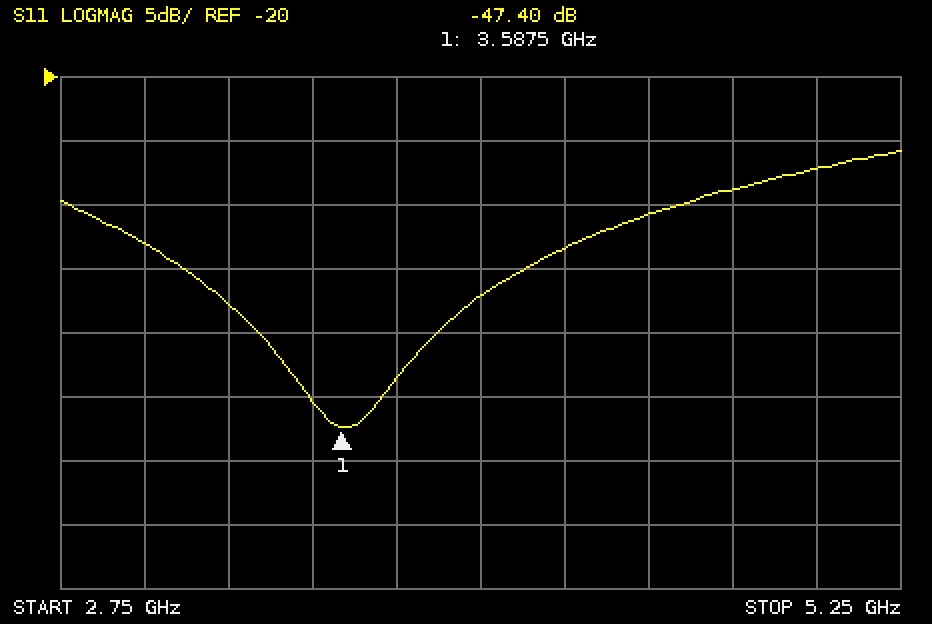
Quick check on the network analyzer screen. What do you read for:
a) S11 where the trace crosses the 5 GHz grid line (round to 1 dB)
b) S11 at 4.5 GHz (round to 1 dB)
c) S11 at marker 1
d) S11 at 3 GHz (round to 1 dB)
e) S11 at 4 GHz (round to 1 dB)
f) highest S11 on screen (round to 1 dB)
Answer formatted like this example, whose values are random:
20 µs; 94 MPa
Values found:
-27 dB; -31 dB; -47.40 dB; -33 dB; -37 dB; -26 dB
